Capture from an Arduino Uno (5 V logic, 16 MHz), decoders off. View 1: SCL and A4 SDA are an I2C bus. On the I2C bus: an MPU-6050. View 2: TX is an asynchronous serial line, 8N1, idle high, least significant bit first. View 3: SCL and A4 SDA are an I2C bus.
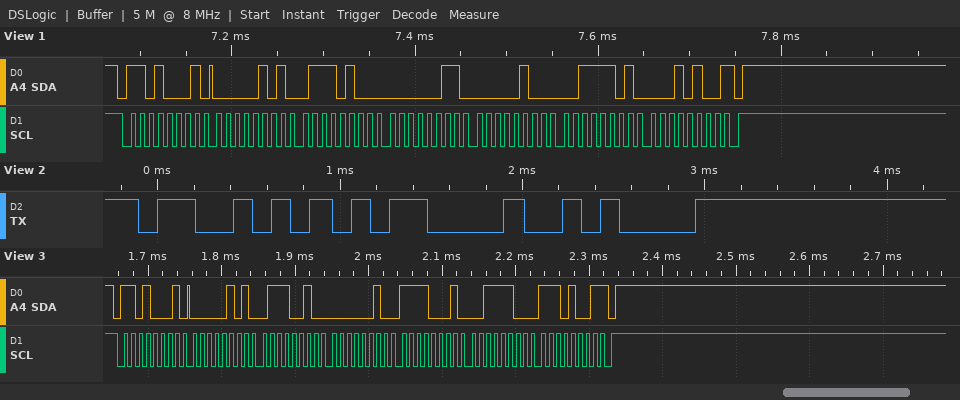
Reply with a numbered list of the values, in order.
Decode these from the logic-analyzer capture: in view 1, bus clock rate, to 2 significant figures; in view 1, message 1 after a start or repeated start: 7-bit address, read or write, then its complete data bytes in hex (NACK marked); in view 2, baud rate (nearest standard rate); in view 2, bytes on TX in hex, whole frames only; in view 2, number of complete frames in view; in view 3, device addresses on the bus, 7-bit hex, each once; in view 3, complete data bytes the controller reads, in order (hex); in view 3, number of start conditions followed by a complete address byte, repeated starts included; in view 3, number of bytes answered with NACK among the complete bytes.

1. 100 kHz
2. 0x68 read: 05 74 03 04 3D 14 NACK
3. 9600 baud
4. 0x53 0x0D 0x0A
5. 3
6. 0x68
7. 05 72 02 F1 3C E9
8. 1
9. 1
